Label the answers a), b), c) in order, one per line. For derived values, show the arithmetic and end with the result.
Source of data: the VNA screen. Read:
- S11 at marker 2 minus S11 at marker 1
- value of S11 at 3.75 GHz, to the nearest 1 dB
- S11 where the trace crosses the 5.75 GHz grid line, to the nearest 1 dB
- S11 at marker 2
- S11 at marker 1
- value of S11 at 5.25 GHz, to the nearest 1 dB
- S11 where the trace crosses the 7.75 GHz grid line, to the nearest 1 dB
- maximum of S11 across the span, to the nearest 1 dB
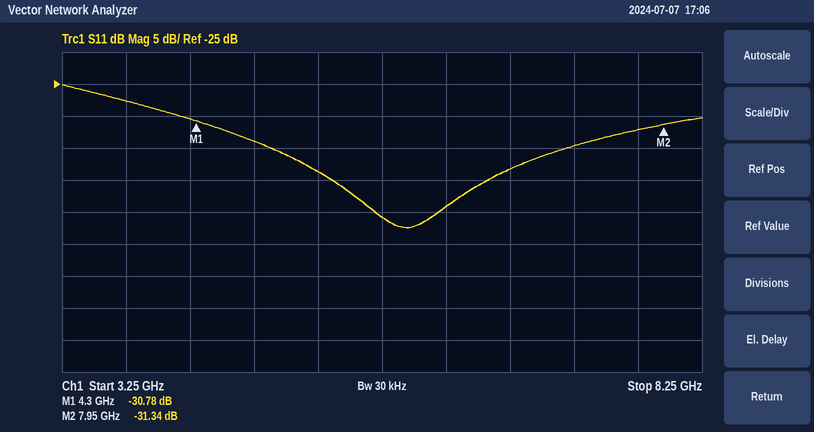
a) -31.34 − (-30.78) = -0.56 dB
b) -28 dB
c) -46 dB
d) -31.34 dB
e) -30.78 dB
f) -39 dB
g) -32 dB
h) -25 dB
